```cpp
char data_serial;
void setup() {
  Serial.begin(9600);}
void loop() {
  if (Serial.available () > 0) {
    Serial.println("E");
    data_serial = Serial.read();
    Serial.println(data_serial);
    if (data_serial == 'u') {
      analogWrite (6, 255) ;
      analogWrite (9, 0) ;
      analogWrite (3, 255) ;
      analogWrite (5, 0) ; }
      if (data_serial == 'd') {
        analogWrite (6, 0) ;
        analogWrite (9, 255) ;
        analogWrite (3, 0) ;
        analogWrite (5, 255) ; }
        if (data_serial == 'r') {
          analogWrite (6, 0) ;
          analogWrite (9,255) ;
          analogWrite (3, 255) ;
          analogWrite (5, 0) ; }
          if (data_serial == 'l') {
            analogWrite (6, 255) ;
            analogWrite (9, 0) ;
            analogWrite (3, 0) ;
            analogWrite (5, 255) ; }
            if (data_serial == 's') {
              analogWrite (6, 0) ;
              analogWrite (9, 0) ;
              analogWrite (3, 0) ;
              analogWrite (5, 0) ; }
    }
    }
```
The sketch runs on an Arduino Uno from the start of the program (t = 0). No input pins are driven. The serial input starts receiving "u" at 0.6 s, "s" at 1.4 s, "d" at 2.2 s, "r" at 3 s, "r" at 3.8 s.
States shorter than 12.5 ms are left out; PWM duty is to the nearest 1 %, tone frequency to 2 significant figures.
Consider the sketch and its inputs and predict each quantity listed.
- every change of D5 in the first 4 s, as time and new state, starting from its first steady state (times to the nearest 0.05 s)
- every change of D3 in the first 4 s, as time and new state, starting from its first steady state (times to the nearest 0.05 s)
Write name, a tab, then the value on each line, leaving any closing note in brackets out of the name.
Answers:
every change of D5 in the first 4 s, as time and new state, starting from its first steady state	0.6 s low; 2.2 s high; 3 s low
every change of D3 in the first 4 s, as time and new state, starting from its first steady state	0.6 s high; 1.4 s low; 3 s high
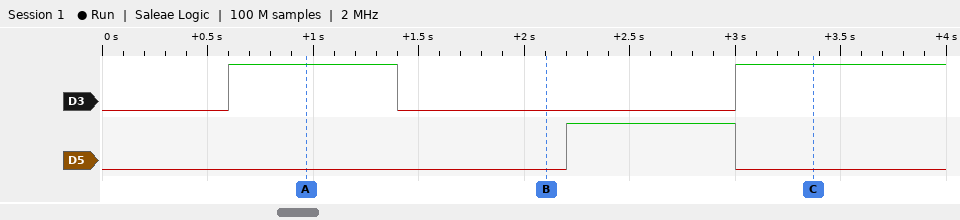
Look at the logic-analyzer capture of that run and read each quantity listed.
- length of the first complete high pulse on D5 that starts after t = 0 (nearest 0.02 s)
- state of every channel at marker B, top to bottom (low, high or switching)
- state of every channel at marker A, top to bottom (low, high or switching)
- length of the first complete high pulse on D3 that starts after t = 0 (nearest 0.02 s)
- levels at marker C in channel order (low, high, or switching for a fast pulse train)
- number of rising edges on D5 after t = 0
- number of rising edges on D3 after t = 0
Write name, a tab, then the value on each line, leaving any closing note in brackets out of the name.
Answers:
length of the first complete high pulse on D5 that starts after t = 0	0.80 s
state of every channel at marker B, top to bottom	D3 low, D5 low
state of every channel at marker A, top to bottom	D3 high, D5 low
length of the first complete high pulse on D3 that starts after t = 0	0.80 s
levels at marker C in channel order	D3 high, D5 low
number of rising edges on D5 after t = 0	1
number of rising edges on D3 after t = 0	2
